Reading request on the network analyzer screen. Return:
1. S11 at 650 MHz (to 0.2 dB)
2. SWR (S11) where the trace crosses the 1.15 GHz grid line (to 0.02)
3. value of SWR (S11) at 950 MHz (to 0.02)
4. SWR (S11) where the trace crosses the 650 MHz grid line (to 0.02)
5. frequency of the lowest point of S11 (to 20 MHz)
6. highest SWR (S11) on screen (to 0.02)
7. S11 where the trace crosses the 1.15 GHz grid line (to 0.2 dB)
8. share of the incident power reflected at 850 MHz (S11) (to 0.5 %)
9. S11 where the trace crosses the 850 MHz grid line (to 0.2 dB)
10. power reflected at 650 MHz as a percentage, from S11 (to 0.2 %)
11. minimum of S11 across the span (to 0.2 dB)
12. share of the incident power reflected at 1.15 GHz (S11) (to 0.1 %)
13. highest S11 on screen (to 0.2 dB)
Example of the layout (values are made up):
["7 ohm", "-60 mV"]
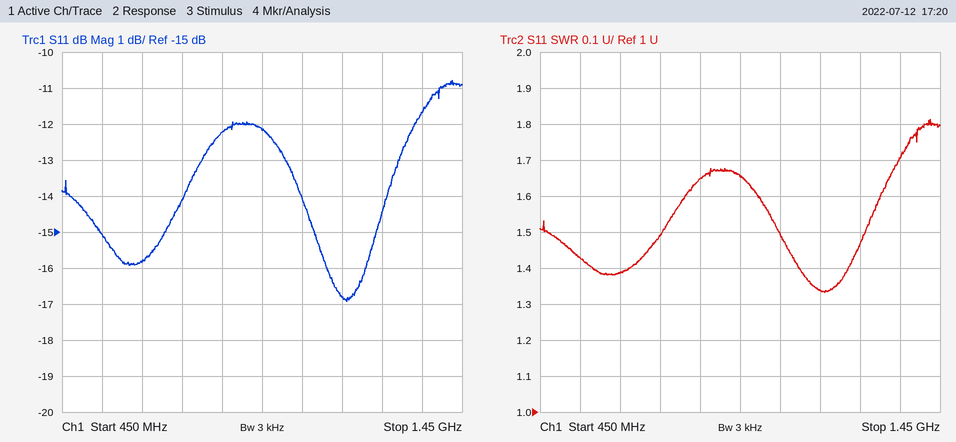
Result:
["-15.8 dB", "1.34", "1.66", "1.38", "1.16 GHz", "1.82", "-16.8 dB", "6.0 %", "-12.2 dB", "2.6 %", "-17.0 dB", "2.1 %", "-10.8 dB"]
